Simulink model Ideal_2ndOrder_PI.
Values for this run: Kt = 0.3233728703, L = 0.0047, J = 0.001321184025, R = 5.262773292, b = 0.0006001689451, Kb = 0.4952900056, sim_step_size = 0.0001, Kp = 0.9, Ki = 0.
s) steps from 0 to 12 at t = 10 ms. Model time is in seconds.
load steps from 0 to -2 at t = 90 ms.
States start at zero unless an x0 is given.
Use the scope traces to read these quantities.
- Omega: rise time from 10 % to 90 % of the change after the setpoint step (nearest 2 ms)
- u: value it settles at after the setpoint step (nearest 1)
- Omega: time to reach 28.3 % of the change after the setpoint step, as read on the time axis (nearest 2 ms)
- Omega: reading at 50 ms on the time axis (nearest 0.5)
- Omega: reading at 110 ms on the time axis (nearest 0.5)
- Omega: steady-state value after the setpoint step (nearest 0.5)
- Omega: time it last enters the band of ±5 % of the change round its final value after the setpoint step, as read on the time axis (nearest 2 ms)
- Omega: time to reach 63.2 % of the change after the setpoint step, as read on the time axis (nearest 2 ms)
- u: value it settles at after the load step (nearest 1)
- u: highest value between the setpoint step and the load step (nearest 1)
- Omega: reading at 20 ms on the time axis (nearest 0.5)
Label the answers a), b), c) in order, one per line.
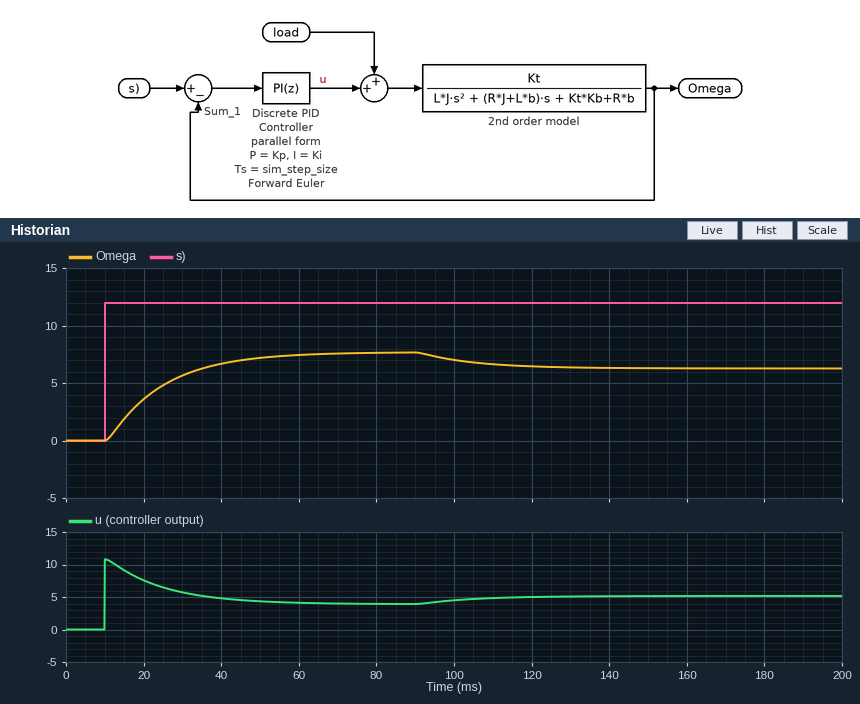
a) 32 ms
b) 4
c) 16 ms
d) 7.0
e) 6.5
f) 7.5
g) 54 ms
h) 26 ms
i) 5
j) 11
k) 3.5
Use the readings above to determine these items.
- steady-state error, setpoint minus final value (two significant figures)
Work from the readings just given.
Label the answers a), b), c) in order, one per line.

a) 4.5
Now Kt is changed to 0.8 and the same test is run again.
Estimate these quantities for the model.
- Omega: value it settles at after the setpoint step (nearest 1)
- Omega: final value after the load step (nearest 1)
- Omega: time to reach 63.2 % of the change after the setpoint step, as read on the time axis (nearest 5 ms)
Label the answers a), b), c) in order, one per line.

a) 8
b) 6
c) 15 ms
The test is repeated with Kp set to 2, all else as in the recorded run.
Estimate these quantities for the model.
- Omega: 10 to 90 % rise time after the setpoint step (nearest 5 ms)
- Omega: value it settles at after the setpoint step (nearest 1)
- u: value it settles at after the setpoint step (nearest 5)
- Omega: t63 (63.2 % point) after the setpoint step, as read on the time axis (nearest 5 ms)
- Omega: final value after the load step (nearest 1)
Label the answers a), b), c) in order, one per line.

a) 15 ms
b) 10
c) 5
d) 20 ms
e) 9
